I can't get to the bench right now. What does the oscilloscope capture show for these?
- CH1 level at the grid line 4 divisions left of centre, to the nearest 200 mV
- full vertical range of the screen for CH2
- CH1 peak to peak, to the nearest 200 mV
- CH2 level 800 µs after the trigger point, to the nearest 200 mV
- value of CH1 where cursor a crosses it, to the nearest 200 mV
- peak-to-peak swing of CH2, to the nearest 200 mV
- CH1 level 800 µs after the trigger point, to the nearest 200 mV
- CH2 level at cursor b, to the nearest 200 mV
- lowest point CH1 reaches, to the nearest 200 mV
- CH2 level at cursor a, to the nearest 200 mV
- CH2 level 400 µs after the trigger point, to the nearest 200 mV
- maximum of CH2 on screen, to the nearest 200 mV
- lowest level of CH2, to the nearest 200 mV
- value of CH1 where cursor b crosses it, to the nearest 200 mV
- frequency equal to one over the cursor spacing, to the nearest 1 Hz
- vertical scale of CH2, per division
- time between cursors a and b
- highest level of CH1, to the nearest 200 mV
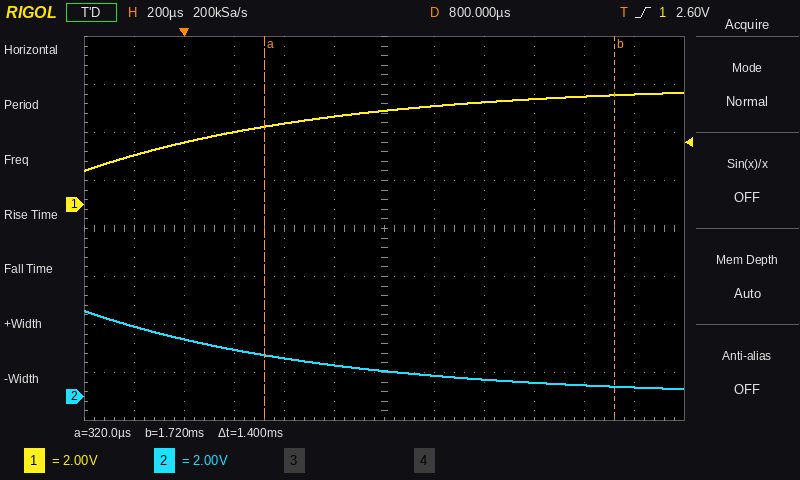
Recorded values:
2.6 V
16 V
3.2 V
1.0 V
3.2 V
3.2 V
4.0 V
400 mV
1.4 V
1.8 V
1.6 V
3.6 V
400 mV
4.6 V
714 Hz
2 V
1.4 ms
4.6 V
